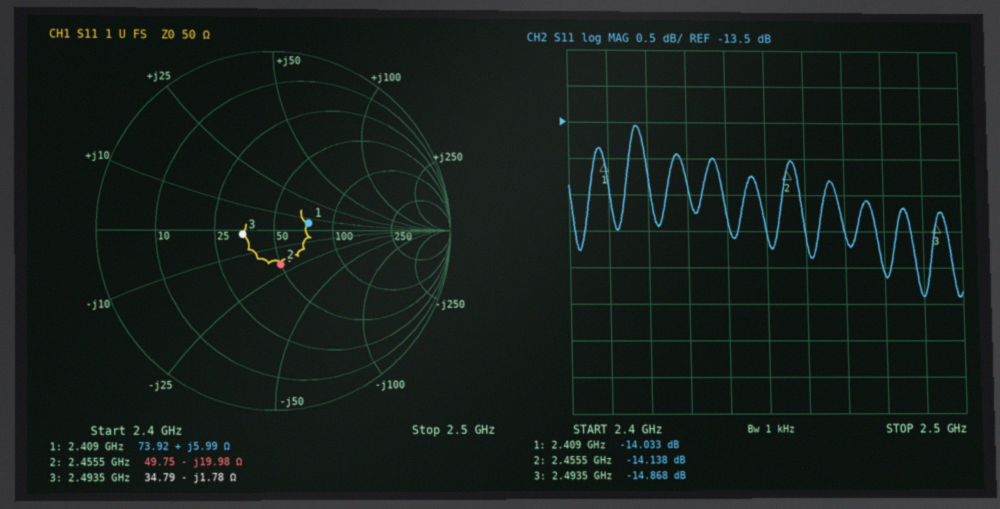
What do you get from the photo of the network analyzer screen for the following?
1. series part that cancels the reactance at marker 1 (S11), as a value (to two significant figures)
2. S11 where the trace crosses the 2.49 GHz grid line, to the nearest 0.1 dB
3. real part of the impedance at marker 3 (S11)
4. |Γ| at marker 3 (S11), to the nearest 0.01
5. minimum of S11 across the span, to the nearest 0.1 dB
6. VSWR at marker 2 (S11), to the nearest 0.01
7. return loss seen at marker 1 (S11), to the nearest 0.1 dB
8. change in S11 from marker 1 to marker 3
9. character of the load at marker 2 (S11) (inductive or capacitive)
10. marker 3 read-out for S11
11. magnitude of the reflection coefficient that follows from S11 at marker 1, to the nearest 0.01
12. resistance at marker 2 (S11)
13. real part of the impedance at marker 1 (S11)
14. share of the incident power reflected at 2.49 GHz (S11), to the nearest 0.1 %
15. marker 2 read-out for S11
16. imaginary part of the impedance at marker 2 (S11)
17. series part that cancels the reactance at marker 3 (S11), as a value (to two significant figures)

11 pF
-15.9 dB
34.79 Ω
0.18
-15.9 dB
1.49
14.0 dB
-0.835 dB
capacitive
-14.868 dB
0.20
49.75 Ω
73.92 Ω
2.6 %
-14.138 dB
-19.98 Ω
110 pH
